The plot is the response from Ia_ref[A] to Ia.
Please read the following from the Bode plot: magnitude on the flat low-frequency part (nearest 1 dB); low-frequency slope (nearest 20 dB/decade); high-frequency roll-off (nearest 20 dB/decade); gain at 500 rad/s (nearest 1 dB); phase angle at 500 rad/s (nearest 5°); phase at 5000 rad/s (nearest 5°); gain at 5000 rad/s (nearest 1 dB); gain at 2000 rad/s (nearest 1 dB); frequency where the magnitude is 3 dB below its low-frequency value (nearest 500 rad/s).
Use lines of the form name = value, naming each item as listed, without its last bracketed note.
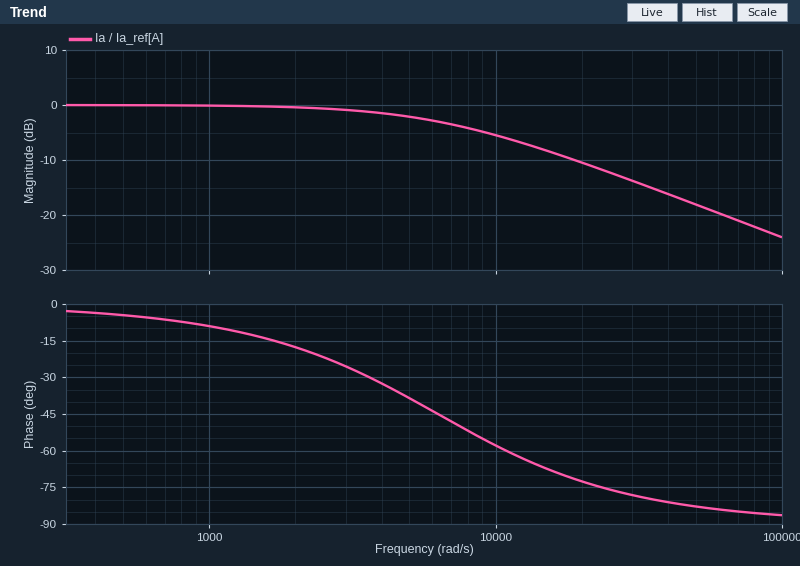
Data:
magnitude on the flat low-frequency part = 0 dB
low-frequency slope = 0 dB/decade
high-frequency roll-off = -20 dB/decade
gain at 500 rad/s = 0 dB
phase angle at 500 rad/s = -5°
phase at 5000 rad/s = -40°
gain at 5000 rad/s = -2 dB
gain at 2000 rad/s = 0 dB
frequency where the magnitude is 3 dB below its low-frequency value = 6500 rad/s
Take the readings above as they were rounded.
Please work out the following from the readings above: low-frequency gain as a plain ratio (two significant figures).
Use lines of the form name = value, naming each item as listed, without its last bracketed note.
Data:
low-frequency gain as a plain ratio = 1.0
